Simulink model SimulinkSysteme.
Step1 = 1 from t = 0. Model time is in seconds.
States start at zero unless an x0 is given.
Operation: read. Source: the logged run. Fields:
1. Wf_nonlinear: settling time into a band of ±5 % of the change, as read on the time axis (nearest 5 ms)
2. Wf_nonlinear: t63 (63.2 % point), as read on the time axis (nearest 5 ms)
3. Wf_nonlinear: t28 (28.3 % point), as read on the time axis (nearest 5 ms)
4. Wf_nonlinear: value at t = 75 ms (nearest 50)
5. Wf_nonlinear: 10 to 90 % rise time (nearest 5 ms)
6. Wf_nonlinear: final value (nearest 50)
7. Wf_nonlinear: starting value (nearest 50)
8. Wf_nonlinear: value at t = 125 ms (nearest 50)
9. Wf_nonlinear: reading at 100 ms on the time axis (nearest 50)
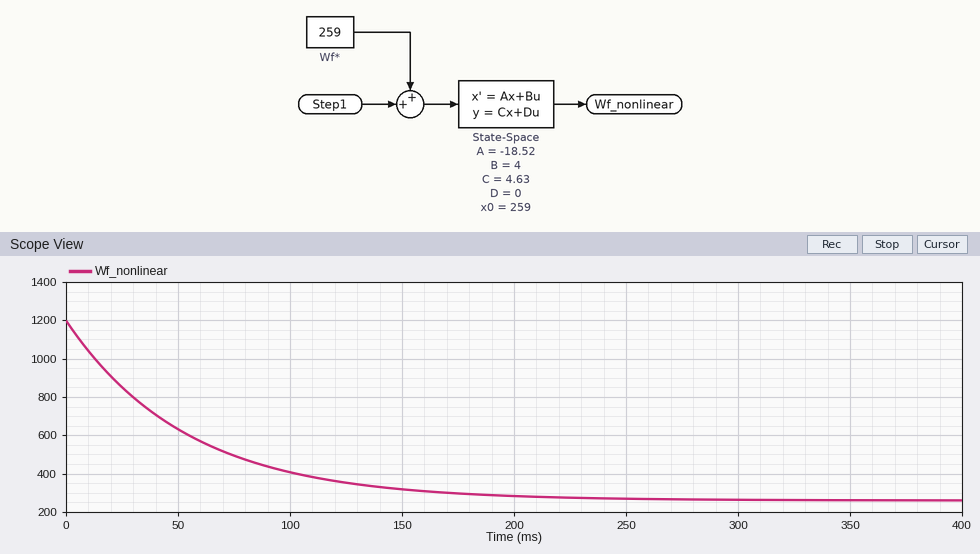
160 ms
55 ms
20 ms
500
120 ms
250
1200
350
400
